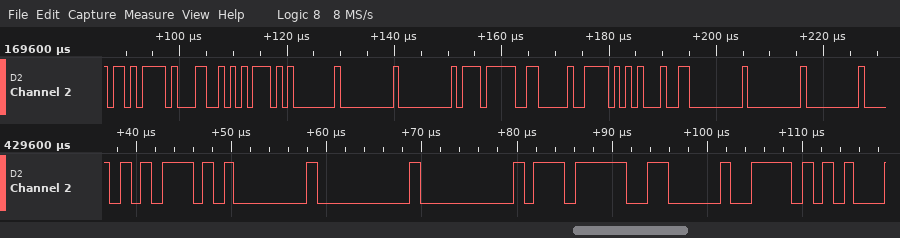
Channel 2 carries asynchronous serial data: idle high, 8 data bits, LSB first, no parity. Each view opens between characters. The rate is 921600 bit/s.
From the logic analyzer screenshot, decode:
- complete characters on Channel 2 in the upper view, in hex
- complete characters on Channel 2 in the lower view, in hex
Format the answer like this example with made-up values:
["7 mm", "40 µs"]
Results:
["EB, 31, 75, 01, 00, 00, F7, 06, 5E, 91, 00, 00, 00", "75, 01, 00, 00, F7, 06, 5E"]
